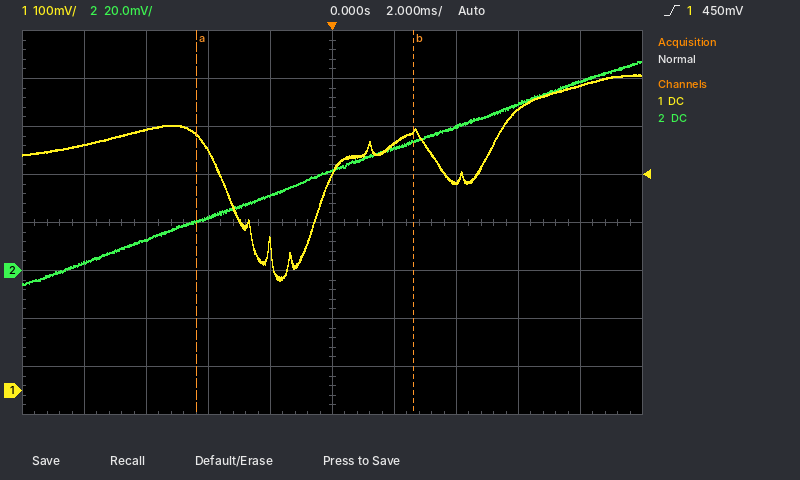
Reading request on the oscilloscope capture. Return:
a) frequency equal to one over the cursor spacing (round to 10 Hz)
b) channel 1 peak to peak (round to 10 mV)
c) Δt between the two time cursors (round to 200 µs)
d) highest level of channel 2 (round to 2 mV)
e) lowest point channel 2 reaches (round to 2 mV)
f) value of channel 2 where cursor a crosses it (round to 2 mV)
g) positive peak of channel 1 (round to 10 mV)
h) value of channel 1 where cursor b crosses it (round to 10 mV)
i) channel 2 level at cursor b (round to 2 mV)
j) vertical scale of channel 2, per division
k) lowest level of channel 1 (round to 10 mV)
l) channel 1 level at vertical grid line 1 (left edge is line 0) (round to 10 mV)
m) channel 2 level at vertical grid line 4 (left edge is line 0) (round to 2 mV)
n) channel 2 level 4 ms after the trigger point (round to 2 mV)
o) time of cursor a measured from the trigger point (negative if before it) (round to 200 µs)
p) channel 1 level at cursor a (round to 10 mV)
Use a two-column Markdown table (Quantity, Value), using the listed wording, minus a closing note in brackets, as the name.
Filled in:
| Quantity | Value |
|---|---|
| frequency equal to one over the cursor spacing | 140 Hz |
| channel 1 peak to peak | 430 mV |
| Δt between the two time cursors | 7.0 ms |
| highest level of channel 2 | 88 mV |
| lowest point channel 2 reaches | -6 mV |
| value of channel 2 where cursor a crosses it | 20 mV |
| positive peak of channel 1 | 660 mV |
| value of channel 1 where cursor b crosses it | 540 mV |
| channel 2 level at cursor b | 54 mV |
| vertical scale of channel 2, per division | 20 mV |
| lowest level of channel 1 | 230 mV |
| channel 1 level at vertical grid line 1 (left edge is line 0) | 510 mV |
| channel 2 level at vertical grid line 4 (left edge is line 0) | 32 mV |
| channel 2 level 4 ms after the trigger point | 60 mV |
| time of cursor a measured from the trigger point (negative if before it) | -4.4 ms |
| channel 1 level at cursor a | 530 mV |
